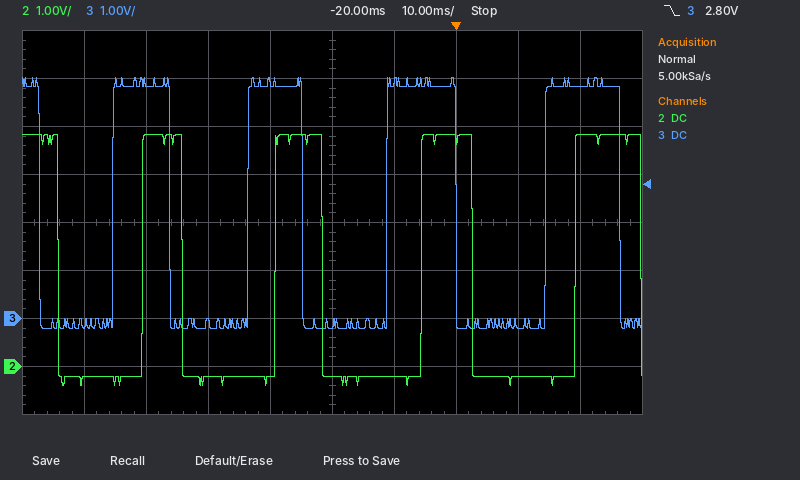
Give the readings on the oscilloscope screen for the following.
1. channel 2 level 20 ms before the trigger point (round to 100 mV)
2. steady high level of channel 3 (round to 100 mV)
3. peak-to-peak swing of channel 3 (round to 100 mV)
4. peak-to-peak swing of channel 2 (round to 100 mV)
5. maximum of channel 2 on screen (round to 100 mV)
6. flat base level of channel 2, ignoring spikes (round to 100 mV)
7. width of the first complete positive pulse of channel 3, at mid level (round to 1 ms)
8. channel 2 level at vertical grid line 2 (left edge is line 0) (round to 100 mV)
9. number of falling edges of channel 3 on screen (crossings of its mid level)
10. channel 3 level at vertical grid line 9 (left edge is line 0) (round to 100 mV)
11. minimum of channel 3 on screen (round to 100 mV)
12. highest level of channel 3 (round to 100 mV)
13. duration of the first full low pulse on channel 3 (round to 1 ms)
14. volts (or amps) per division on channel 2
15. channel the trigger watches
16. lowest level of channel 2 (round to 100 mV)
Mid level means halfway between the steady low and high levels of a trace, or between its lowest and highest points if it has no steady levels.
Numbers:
-200 mV
4.8 V
5.2 V
5.2 V
4.8 V
-200 mV
9 ms
4.8 V
5
4.8 V
-200 mV
5.0 V
12 ms
1 V
channel 3
-400 mV
